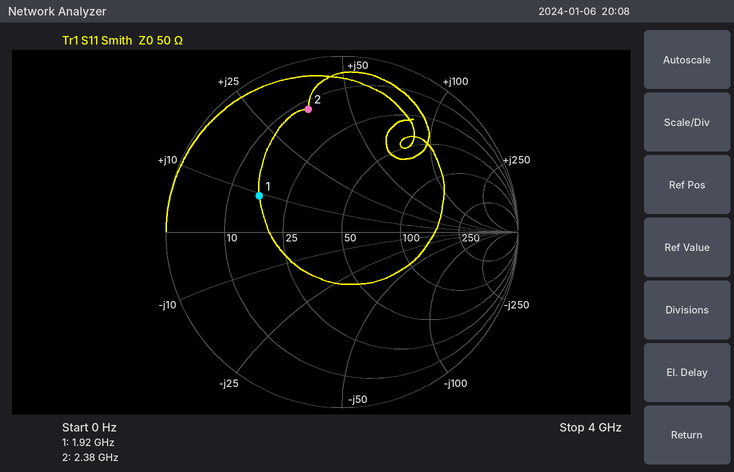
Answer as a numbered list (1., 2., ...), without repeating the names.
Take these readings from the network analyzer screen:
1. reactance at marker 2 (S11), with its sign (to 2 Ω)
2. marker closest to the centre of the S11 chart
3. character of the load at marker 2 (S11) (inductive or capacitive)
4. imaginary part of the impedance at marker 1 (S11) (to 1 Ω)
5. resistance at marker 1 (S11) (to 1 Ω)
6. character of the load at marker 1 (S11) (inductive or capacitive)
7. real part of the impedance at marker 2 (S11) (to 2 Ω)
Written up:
1. +36 Ω
2. marker 1
3. inductive
4. +9 Ω
5. 17 Ω
6. inductive
7. 12 Ω
